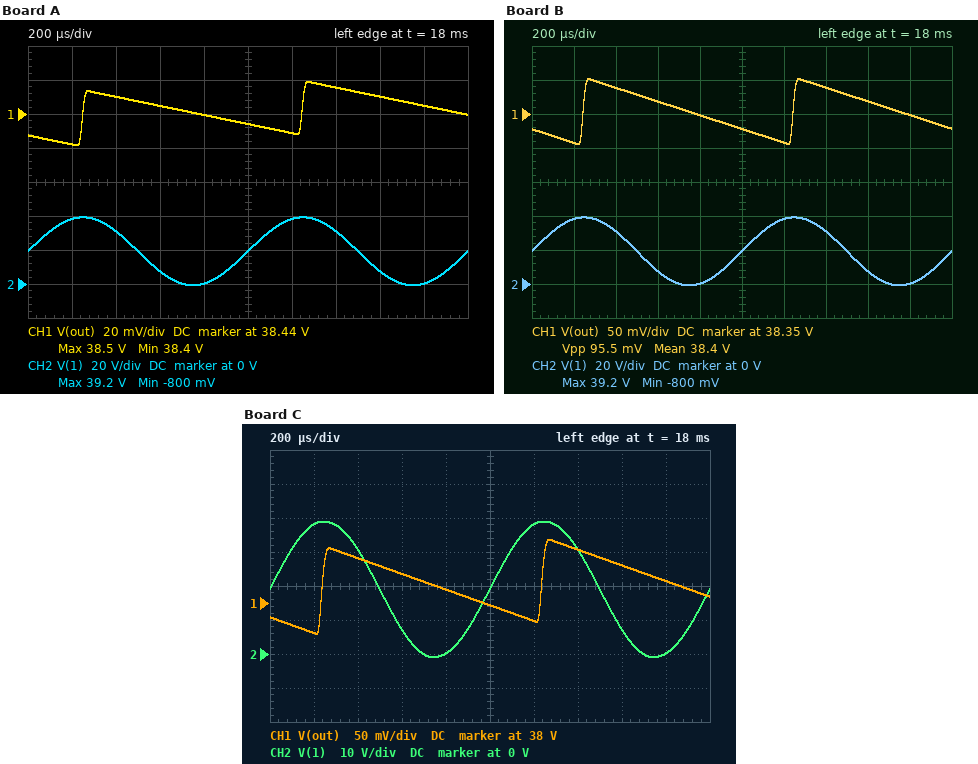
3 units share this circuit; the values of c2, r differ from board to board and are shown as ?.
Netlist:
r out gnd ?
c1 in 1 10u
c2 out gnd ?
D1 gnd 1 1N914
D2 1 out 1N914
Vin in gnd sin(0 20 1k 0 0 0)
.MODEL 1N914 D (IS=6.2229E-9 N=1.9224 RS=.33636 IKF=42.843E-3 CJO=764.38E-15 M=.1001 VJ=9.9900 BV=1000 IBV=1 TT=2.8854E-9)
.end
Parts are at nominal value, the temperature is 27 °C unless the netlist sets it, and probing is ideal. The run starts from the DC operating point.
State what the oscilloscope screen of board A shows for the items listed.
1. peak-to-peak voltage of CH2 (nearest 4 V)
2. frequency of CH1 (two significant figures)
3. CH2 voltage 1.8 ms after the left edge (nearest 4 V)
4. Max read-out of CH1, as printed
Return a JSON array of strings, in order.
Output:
["40 V", "1.0 kHz", "0 V", "38.5 V"]
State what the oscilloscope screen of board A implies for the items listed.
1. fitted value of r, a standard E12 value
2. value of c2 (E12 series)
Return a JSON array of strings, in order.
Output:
["120 kΩ", "12 µF"]
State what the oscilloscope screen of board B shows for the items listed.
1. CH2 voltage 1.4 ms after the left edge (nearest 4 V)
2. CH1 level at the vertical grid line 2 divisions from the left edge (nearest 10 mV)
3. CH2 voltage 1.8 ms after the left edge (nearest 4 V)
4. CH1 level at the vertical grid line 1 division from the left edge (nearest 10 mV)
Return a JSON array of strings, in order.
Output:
["32 V", "38.39 V", "0 V", "38.31 V"]
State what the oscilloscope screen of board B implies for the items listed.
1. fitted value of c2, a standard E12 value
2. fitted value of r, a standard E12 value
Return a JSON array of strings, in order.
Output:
["6.8 µF", "56 kΩ"]
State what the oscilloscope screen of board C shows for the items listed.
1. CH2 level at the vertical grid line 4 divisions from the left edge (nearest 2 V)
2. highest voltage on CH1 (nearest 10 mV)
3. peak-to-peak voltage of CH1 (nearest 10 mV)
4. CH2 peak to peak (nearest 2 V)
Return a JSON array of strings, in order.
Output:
["0 V", "38.09 V", "140 mV", "40 V"]
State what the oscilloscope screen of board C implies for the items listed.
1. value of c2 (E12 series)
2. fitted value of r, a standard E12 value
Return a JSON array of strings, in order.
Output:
["22 µF", "15 kΩ"]
